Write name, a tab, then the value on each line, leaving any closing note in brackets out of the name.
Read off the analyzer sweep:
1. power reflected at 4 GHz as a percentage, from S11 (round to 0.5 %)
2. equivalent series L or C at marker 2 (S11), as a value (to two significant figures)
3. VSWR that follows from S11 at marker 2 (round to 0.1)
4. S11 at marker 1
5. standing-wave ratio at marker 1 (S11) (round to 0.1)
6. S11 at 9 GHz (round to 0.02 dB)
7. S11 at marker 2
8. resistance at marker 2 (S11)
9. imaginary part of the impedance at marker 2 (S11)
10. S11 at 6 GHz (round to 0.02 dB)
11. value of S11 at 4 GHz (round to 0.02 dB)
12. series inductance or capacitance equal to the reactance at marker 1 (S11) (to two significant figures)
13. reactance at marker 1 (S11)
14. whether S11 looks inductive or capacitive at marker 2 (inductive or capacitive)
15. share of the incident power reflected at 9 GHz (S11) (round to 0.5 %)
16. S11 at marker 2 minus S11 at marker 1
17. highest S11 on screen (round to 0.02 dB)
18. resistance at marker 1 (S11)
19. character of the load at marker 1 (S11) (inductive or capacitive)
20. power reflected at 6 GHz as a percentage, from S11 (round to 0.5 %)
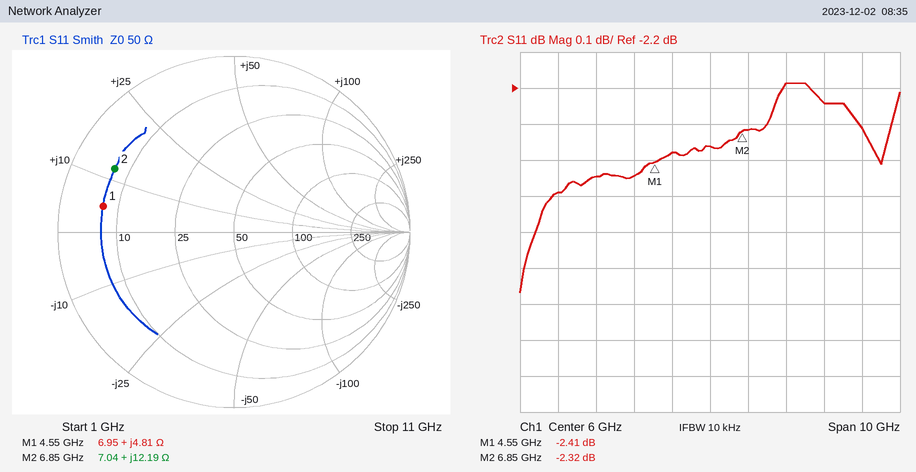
power reflected at 4 GHz as a percentage, from S11	57.0 %
equivalent series L or C at marker 2 (S11), as a value	280 pH
VSWR that follows from S11 at marker 2	7.5
S11 at marker 1	-2.41 dB
standing-wave ratio at marker 1 (S11)	7.3
S11 at 9 GHz	-2.24 dB
S11 at marker 2	-2.32 dB
resistance at marker 2	7.04 Ω
imaginary part of the impedance at marker 2	+12.19 Ω
S11 at 6 GHz	-2.36 dB
value of S11 at 4 GHz	-2.44 dB
series inductance or capacitance equal to the reactance at marker 1 (S11)	170 pH
reactance at marker 1	+4.81 Ω
whether S11 looks inductive or capacitive at marker 2	inductive
share of the incident power reflected at 9 GHz (S11)	59.5 %
S11 at marker 2 minus S11 at marker 1	0.09 dB
highest S11 on screen	-2.18 dB
resistance at marker 1	6.95 Ω
character of the load at marker 1 (S11)	inductive
power reflected at 6 GHz as a percentage, from S11	58.0 %
